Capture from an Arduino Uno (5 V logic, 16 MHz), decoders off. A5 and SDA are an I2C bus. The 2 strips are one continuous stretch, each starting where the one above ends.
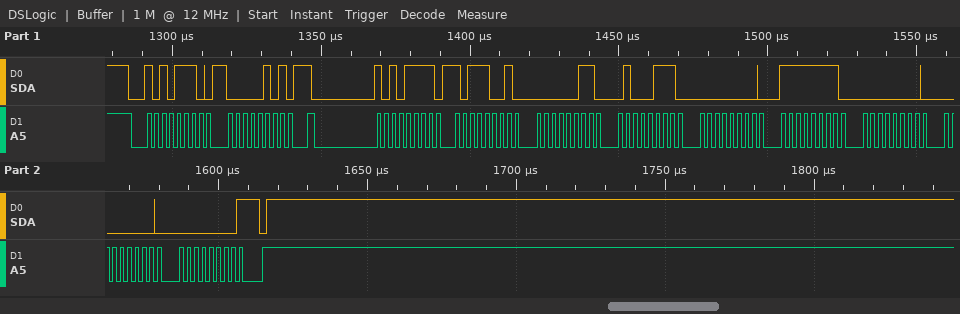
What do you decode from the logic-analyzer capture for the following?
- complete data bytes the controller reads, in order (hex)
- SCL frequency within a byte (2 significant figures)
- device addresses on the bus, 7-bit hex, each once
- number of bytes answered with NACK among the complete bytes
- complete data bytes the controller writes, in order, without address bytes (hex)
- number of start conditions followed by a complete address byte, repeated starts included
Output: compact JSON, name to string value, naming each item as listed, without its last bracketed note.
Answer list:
{"complete data bytes the controller reads, in order": "B9 03 47 00 FF 00 00 00", "SCL frequency within a byte": "400 kHz", "device addresses on the bus, 7-bit hex, each once": "0x57", "number of bytes answered with NACK among the complete bytes": "1", "complete data bytes the controller writes, in order, without address bytes": "05", "number of start conditions followed by a complete address byte, repeated starts included": "2"}
